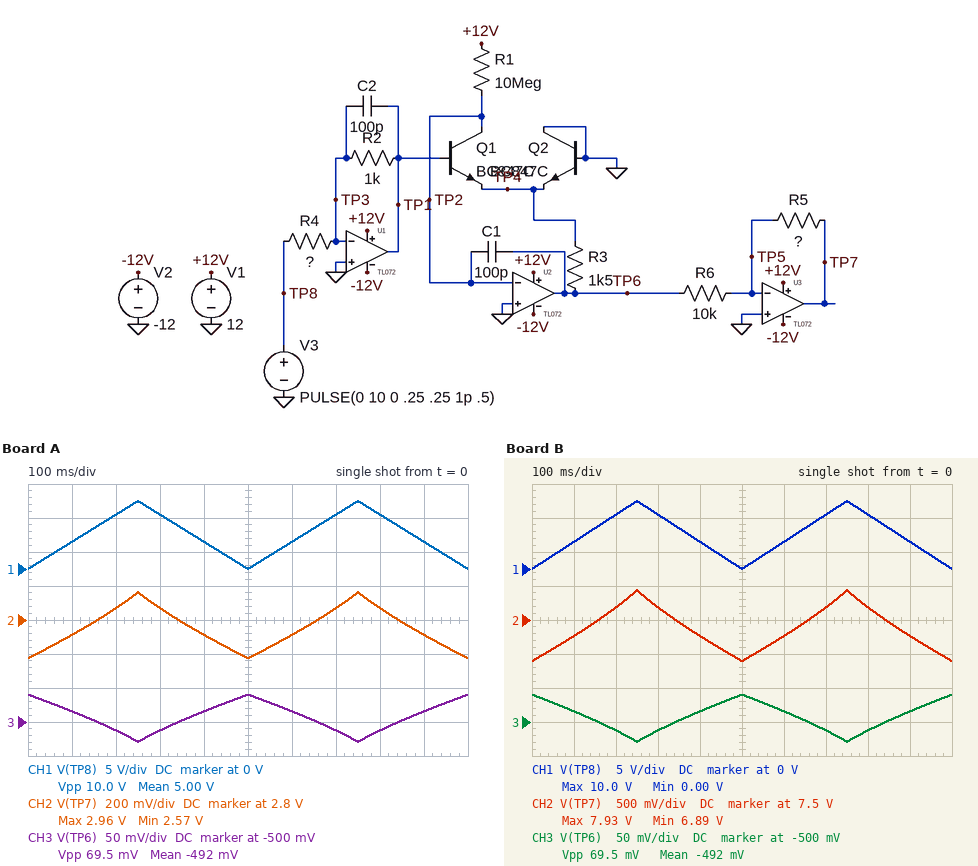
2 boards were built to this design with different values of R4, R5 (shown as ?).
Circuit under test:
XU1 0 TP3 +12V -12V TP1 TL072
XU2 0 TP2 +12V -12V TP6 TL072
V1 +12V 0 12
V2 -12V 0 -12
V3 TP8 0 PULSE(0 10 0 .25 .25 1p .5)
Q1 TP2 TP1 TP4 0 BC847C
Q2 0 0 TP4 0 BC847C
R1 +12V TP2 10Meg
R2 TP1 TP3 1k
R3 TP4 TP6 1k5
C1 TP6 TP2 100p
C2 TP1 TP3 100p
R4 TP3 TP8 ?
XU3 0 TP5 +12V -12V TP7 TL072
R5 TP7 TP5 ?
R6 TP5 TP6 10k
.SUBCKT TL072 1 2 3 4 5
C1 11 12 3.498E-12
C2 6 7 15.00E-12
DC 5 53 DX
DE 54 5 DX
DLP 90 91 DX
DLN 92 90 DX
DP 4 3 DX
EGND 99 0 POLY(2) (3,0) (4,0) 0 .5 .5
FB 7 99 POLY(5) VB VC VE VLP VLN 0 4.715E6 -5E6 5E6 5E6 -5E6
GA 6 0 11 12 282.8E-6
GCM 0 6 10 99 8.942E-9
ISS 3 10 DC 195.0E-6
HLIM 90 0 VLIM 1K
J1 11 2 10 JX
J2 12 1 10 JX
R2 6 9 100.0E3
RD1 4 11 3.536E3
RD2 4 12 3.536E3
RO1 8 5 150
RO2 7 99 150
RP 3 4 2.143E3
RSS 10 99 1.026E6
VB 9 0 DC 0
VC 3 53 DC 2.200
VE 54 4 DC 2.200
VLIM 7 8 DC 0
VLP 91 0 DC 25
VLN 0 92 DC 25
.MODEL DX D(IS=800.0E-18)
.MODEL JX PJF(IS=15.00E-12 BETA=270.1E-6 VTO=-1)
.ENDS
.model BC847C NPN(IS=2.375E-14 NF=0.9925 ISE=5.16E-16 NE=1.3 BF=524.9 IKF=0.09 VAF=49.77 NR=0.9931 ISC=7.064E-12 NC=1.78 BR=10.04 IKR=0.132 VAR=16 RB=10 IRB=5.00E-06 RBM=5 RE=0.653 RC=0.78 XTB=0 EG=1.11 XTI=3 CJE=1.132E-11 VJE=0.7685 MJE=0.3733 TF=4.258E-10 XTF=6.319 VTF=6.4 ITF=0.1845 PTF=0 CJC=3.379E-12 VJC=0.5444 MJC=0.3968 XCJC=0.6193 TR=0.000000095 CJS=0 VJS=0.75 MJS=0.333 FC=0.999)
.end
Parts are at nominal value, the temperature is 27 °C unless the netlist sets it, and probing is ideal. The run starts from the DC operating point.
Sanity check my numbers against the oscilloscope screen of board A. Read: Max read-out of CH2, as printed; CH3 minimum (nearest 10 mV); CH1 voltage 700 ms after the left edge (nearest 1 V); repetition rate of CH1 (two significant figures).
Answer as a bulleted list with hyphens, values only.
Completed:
- 2.96 V
- -530 mV
- 8 V
- 2.0 Hz
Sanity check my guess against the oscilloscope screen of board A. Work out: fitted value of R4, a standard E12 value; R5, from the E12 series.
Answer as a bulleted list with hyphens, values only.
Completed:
- 180 kΩ
- 56 kΩ
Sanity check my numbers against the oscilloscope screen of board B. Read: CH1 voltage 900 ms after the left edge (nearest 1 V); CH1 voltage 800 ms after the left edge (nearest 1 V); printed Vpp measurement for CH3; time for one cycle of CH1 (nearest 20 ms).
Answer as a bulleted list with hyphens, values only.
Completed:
- 4 V
- 8 V
- 69.5 mV
- 500 ms
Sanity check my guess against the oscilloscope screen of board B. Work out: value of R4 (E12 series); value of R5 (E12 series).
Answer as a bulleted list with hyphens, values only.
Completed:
- 180 kΩ
- 150 kΩ
